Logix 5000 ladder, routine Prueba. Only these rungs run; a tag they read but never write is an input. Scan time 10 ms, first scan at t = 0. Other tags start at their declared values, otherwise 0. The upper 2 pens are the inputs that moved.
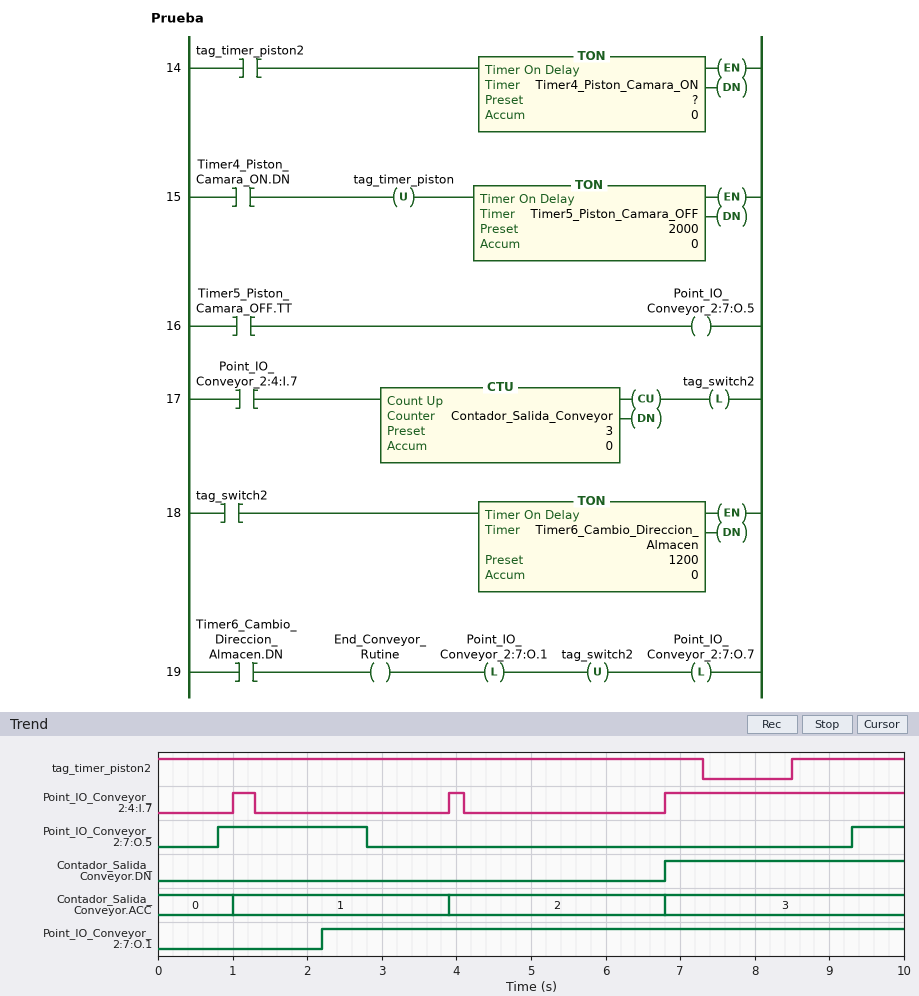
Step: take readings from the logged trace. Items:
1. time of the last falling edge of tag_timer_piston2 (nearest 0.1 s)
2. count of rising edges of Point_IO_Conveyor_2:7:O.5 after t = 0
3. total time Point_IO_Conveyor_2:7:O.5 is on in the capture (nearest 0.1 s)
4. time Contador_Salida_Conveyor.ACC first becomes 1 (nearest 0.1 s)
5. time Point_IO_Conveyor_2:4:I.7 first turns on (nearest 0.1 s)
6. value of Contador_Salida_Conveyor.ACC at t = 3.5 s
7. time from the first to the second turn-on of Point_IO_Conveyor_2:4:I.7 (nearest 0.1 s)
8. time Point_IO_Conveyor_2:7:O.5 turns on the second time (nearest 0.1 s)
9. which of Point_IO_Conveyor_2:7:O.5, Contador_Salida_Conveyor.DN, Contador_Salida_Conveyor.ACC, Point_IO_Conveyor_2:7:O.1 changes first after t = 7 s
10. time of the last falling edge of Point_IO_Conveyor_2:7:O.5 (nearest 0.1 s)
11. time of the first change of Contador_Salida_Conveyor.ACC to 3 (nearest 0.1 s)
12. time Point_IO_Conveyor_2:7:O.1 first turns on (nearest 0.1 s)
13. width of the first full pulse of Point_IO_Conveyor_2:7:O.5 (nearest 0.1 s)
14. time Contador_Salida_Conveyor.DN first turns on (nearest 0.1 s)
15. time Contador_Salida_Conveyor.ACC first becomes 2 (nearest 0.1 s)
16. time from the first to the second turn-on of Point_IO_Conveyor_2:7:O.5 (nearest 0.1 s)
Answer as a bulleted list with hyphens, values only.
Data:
- 7.3 s
- 2
- 2.7 s
- 1.0 s
- 1.0 s
- 1
- 2.9 s
- 9.3 s
- Point_IO_Conveyor_2:7:O.5
- 2.8 s
- 6.8 s
- 2.2 s
- 2.0 s
- 6.8 s
- 3.9 s
- 8.5 s
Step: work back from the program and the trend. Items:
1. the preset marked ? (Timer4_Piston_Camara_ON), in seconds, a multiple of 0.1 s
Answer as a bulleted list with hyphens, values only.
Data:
- 0.8 s
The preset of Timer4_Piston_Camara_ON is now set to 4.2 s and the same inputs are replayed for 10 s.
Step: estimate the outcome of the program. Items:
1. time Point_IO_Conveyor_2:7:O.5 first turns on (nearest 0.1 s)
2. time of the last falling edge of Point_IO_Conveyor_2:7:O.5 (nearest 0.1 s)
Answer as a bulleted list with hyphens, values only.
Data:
- 4.2 s
- 6.2 s
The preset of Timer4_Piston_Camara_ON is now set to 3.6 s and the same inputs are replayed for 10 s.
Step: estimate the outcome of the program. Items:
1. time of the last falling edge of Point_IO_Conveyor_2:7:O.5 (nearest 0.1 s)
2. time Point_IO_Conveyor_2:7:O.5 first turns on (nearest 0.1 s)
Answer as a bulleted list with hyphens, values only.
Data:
- 5.6 s
- 3.6 s
